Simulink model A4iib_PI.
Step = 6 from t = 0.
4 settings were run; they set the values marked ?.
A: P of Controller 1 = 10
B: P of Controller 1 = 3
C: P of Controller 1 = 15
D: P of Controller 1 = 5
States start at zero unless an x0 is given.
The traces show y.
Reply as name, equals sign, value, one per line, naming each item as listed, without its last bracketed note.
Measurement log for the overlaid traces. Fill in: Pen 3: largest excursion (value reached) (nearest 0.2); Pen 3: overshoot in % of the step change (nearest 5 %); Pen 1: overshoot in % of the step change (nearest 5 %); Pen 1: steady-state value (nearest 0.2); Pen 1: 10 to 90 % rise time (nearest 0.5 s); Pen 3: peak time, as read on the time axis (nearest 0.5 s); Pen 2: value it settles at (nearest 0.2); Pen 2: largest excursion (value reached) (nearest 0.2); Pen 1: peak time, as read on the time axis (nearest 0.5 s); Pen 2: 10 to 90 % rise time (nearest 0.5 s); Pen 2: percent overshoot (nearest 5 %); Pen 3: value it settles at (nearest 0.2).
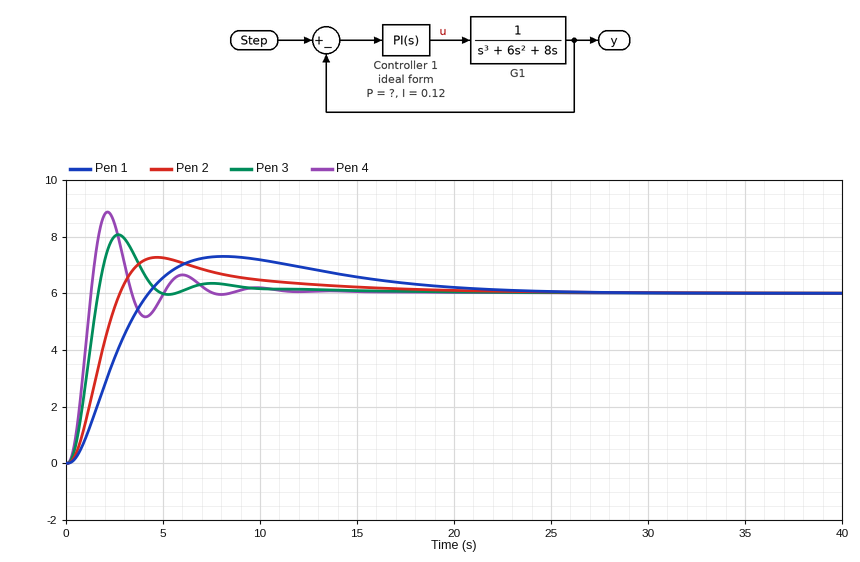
Pen 3: largest excursion (value reached) = 8.0
Pen 3: overshoot in % of the step change = 35 %
Pen 1: overshoot in % of the step change = 20 %
Pen 1: steady-state value = 6.0
Pen 1: 10 to 90 % rise time = 3.0 s
Pen 3: peak time, as read on the time axis = 2.5 s
Pen 2: value it settles at = 6.0
Pen 2: largest excursion (value reached) = 7.2
Pen 1: peak time, as read on the time axis = 8.0 s
Pen 2: 10 to 90 % rise time = 2.0 s
Pen 2: percent overshoot = 20 %
Pen 3: value it settles at = 6.0
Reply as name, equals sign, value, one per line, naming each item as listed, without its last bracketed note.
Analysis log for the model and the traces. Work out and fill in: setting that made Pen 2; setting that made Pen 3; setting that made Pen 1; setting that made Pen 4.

setting that made Pen 2 = D
setting that made Pen 3 = A
setting that made Pen 1 = B
setting that made Pen 4 = C
